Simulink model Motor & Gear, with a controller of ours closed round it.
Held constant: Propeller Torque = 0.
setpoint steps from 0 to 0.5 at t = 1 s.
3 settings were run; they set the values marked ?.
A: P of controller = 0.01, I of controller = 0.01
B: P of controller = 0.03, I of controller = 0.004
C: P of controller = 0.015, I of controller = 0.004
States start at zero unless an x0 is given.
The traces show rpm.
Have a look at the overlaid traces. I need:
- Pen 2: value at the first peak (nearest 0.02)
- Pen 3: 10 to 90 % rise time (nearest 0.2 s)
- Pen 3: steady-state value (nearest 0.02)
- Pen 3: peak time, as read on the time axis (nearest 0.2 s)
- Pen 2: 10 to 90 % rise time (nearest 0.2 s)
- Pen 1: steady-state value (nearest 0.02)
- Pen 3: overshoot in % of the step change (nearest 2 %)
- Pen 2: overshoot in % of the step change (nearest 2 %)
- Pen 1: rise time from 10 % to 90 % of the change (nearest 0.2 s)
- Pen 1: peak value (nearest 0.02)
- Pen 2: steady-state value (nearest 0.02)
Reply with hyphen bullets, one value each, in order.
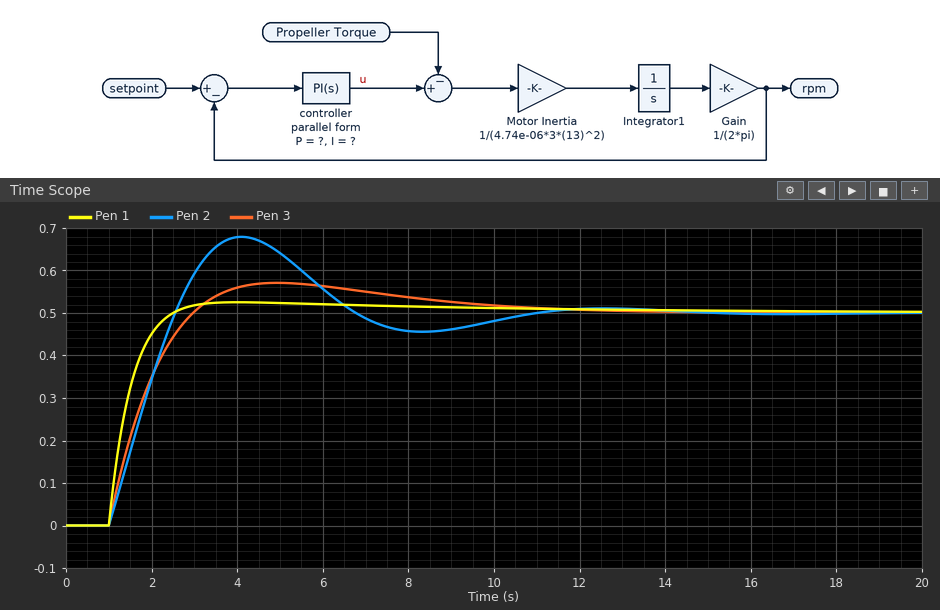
- 0.68
- 1.4 s
- 0.50
- 5.0 s
- 1.2 s
- 0.50
- 14 %
- 36 %
- 1.0 s
- 0.52
- 0.50
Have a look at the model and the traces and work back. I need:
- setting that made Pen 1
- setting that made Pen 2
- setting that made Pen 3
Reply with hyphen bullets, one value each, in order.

- B
- A
- C
